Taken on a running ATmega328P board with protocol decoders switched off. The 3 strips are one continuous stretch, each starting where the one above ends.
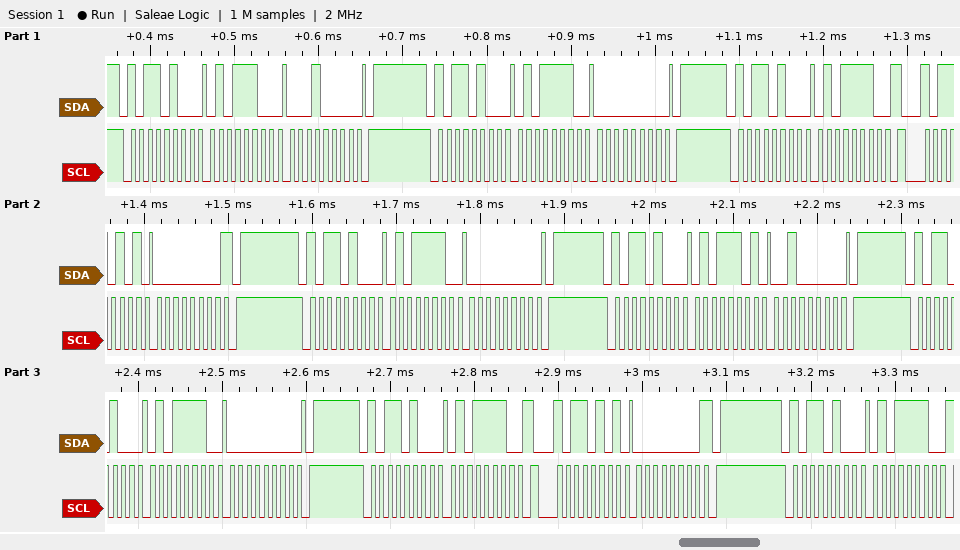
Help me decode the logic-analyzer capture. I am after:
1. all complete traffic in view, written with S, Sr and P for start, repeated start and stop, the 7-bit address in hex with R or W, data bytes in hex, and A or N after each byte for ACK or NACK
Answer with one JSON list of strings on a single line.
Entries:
["S 5AW A 5C A 10 A P S 5AW A 5E A 00 A P S 5AW A 5E A Sr 5AR A 00 N P S 5AW A 5E A 00 A P S 5AW A 5D A 20 A P S 5AW A 5E A 00 A P S 5AW A 5E A Sr 5AR A 00 N P S 5AW A 5E A"]
